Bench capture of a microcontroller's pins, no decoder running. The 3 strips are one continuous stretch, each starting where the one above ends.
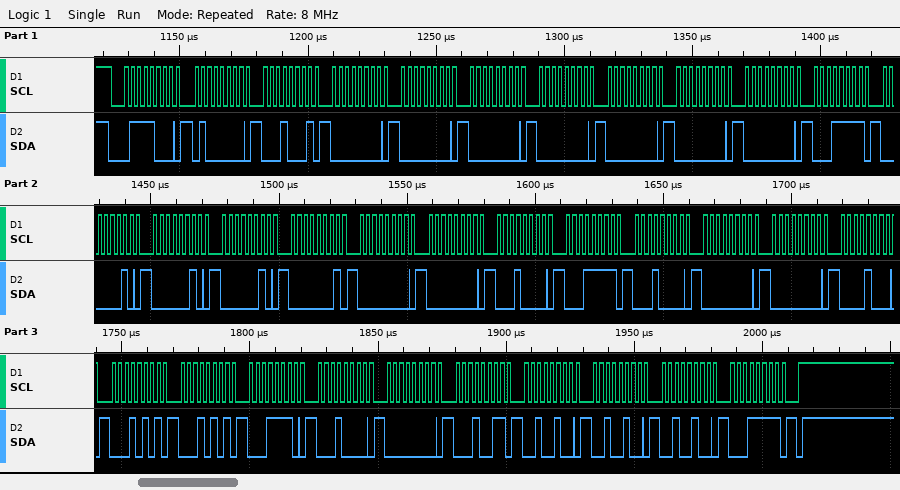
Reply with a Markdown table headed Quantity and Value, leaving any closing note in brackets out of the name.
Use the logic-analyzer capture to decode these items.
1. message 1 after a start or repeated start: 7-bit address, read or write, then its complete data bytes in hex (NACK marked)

| Quantity | Value |
|---|---|
| message 1 after a start or repeated start: 7-bit address, read or write, then its complete data bytes in hex | 0x3C write: 40 11 00 00 00 00 00 00 00 1F 02 02 02 01 00 00 10 1F 10 00 00 08 15 15 1E 10 00 13 24 24 24 1F |
